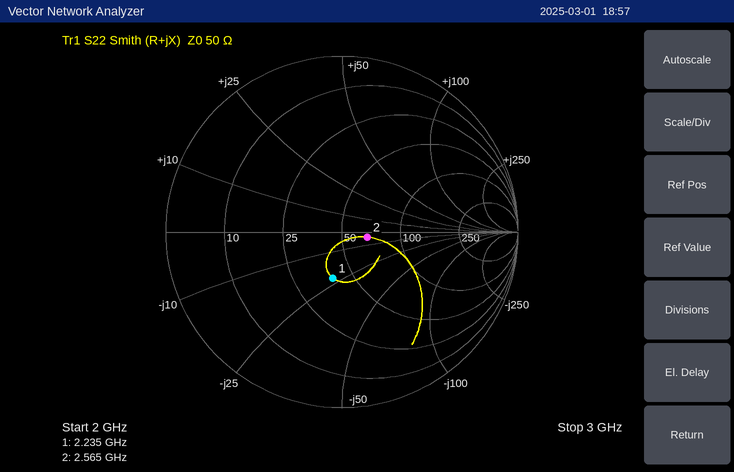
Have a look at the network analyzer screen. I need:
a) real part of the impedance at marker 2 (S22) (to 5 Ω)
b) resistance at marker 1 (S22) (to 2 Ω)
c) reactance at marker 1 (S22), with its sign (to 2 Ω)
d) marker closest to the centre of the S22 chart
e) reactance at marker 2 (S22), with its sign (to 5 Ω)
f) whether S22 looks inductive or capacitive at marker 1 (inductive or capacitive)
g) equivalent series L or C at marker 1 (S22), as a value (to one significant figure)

65 Ω
40 Ω
-22 Ω
marker 2
-5 Ω
capacitive
3 pF
